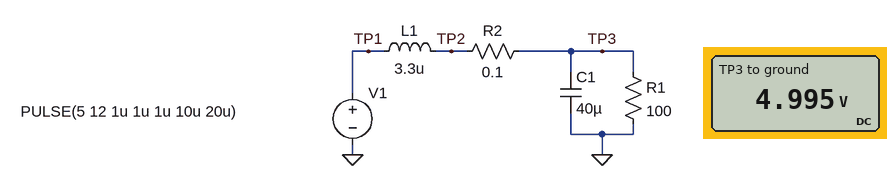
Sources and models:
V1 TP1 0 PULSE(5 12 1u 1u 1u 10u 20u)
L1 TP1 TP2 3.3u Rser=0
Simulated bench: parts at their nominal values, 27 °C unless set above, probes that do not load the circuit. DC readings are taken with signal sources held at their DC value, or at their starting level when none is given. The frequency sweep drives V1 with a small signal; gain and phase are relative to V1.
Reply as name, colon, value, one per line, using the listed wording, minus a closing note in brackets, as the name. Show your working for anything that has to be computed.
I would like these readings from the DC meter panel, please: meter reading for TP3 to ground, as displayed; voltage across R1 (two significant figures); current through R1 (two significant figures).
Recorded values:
meter reading for TP3 to ground, as displayed: 4.995 V
voltage across R1: 4.995 V = 5.0 V
current through R1: (4.995 V) / 100 Ω = 50 mA
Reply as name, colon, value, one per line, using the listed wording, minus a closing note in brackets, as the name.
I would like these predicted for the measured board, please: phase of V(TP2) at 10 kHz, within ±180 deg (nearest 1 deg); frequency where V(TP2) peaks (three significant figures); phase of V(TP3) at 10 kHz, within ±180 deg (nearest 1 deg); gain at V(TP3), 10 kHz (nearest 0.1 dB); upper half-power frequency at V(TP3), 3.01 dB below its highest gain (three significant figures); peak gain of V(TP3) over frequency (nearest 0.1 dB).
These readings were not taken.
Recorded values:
phase of V(TP2) at 10 kHz, within ±180 deg: -14 deg
frequency where V(TP2) peaks: 13.5 kHz
phase of V(TP3) at 10 kHz, within ±180 deg: -28 deg
gain at V(TP3), 10 kHz: 5.3 dB
upper half-power frequency at V(TP3), 3.01 dB below its highest gain: 15.7 kHz
peak gain of V(TP3) over frequency: 9.2 dB
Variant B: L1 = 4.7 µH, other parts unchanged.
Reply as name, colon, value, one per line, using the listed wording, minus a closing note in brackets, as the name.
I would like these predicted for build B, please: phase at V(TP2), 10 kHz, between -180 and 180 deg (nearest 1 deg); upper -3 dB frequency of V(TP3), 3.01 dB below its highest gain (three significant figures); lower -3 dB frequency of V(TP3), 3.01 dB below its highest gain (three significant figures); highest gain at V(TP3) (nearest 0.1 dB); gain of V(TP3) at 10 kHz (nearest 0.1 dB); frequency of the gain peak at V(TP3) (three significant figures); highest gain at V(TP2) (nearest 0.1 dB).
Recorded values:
phase at V(TP2), 10 kHz, between -180 and 180 deg: -30 deg
upper -3 dB frequency of V(TP3), 3.01 dB below its highest gain: 13.0 kHz
lower -3 dB frequency of V(TP3), 3.01 dB below its highest gain: 9.47 kHz
highest gain at V(TP3): 10.7 dB
gain of V(TP3) at 10 kHz: 8.8 dB
frequency of the gain peak at V(TP3): 11.4 kHz
highest gain at V(TP2): 11.0 dB
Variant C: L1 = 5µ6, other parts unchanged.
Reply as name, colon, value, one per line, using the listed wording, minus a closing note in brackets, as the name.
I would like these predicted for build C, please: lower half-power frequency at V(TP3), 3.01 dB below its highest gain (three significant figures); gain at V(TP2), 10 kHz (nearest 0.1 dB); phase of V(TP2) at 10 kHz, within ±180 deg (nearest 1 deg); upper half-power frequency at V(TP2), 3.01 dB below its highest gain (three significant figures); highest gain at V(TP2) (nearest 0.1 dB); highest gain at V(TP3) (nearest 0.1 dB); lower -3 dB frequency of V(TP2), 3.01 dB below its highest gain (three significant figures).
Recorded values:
lower half-power frequency at V(TP3), 3.01 dB below its highest gain: 8.87 kHz
gain at V(TP2), 10 kHz: 11.3 dB
phase of V(TP2) at 10 kHz, within ±180 deg: -51 deg
upper half-power frequency at V(TP2), 3.01 dB below its highest gain: 11.8 kHz
highest gain at V(TP2): 11.7 dB
highest gain at V(TP3): 11.4 dB
lower -3 dB frequency of V(TP2), 3.01 dB below its highest gain: 8.90 kHz
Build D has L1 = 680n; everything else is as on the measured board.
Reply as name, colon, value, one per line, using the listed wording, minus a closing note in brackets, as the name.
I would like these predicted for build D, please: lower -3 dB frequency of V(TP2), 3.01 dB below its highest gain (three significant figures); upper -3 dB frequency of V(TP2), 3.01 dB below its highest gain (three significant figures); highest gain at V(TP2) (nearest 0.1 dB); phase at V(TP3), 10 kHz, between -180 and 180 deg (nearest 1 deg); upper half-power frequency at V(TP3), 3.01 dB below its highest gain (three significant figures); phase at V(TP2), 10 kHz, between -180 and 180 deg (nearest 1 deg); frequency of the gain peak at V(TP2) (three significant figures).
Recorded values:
lower -3 dB frequency of V(TP2), 3.01 dB below its highest gain: 13.2 kHz
upper -3 dB frequency of V(TP2), 3.01 dB below its highest gain: 39.0 kHz
highest gain at V(TP2): 4.6 dB
phase at V(TP3), 10 kHz, between -180 and 180 deg: -16 deg
upper half-power frequency at V(TP3), 3.01 dB below its highest gain: 36.3 kHz
phase at V(TP2), 10 kHz, between -180 and 180 deg: -2 deg
frequency of the gain peak at V(TP2): 27.4 kHz
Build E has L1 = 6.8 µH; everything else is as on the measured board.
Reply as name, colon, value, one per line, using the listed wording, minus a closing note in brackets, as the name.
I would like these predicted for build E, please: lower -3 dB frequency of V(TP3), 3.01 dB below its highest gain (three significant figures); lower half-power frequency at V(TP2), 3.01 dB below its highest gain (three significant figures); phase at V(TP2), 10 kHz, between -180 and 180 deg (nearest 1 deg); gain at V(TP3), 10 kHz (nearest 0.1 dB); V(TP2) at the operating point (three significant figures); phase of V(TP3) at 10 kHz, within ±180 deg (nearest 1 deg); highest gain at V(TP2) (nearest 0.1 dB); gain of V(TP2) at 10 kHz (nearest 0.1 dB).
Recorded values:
lower -3 dB frequency of V(TP3), 3.01 dB below its highest gain: 8.22 kHz
lower half-power frequency at V(TP2), 3.01 dB below its highest gain: 8.24 kHz
phase at V(TP2), 10 kHz, between -180 and 180 deg: -92 deg
gain at V(TP3), 10 kHz: 11.5 dB
V(TP2) at the operating point: 5.00 V
phase of V(TP3) at 10 kHz, within ±180 deg: -106 deg
highest gain at V(TP2): 12.5 dB
gain of V(TP2) at 10 kHz: 11.8 dB
